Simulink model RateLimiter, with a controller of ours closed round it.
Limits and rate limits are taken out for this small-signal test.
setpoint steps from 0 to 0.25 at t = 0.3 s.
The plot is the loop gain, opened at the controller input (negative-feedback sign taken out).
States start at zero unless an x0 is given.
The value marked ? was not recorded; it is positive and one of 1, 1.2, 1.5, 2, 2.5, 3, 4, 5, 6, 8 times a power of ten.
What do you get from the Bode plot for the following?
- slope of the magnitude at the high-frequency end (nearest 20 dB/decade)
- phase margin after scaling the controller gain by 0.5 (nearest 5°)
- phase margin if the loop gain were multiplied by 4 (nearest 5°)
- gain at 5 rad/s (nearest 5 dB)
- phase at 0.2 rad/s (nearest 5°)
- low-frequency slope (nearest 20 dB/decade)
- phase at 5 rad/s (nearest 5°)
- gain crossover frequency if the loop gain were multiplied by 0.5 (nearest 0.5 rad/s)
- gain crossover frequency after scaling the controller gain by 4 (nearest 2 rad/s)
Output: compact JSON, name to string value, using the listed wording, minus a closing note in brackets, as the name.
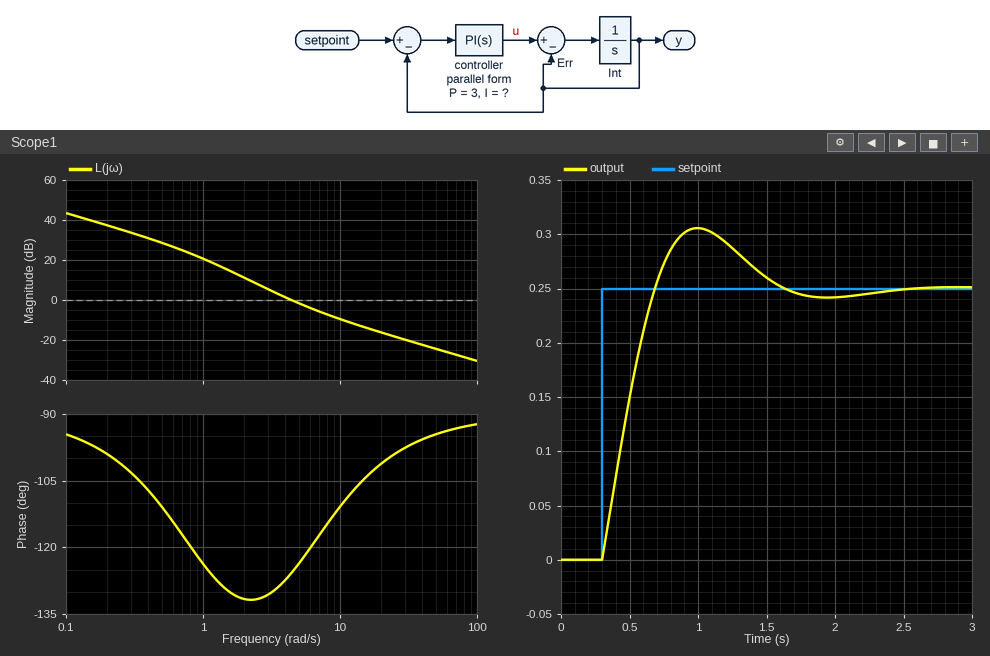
{"slope of the magnitude at the high-frequency end": "-20 dB/decade", "phase margin after scaling the controller gain by 0.5": "50°", "phase margin if the loop gain were multiplied by 4": "75°", "gain at 5 rad/s": "0 dB", "phase at 0.2 rad/s": "-100°", "low-frequency slope": "-20 dB/decade", "phase at 5 rad/s": "-125°", "gain crossover frequency if the loop gain were multiplied by 0.5": "3.0 rad/s", "gain crossover frequency after scaling the controller gain by 4": "12 rad/s"}
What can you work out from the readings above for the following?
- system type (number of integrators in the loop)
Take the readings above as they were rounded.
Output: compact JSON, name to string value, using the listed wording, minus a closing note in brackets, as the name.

{"system type": "1"}
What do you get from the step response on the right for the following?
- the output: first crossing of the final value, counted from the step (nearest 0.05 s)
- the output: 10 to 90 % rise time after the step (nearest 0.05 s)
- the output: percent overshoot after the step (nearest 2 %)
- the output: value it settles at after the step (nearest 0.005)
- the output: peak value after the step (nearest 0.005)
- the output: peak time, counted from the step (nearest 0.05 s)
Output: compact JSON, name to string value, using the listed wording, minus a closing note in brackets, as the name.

{"the output: first crossing of the final value, counted from the step": "0.40 s", "the output: 10 to 90 % rise time after the step": "0.30 s", "the output: percent overshoot after the step": "22 %", "the output: value it settles at after the step": "0.250", "the output: peak value after the step": "0.305", "the output: peak time, counted from the step": "0.70 s"}
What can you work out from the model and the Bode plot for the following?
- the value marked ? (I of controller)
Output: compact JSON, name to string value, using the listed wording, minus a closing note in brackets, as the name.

{"the value marked ?": "15"}
